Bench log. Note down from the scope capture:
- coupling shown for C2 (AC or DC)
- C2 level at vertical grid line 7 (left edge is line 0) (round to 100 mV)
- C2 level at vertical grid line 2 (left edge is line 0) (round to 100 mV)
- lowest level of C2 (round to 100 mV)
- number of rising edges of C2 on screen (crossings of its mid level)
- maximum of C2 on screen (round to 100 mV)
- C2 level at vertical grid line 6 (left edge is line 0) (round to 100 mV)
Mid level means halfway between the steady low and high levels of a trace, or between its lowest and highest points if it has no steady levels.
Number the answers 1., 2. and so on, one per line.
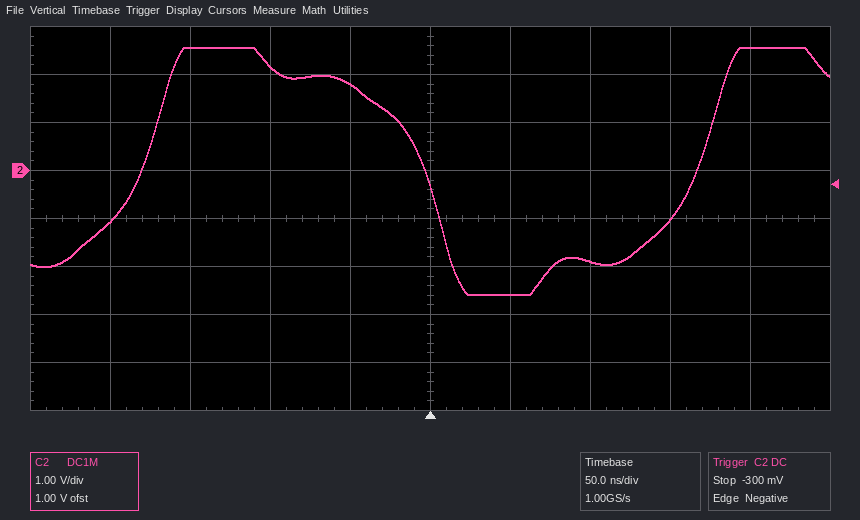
1. DC
2. -1.9 V
3. 2.6 V
4. -2.6 V
5. 2
6. 2.6 V
7. -2.6 V
